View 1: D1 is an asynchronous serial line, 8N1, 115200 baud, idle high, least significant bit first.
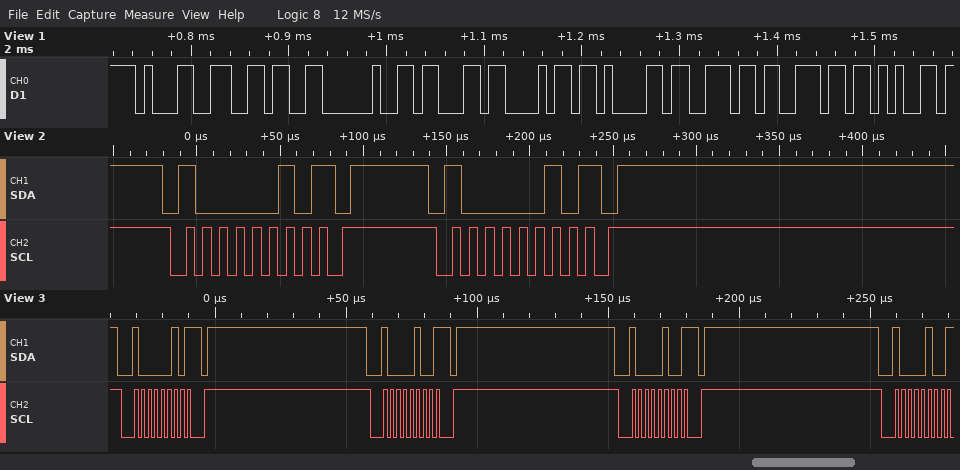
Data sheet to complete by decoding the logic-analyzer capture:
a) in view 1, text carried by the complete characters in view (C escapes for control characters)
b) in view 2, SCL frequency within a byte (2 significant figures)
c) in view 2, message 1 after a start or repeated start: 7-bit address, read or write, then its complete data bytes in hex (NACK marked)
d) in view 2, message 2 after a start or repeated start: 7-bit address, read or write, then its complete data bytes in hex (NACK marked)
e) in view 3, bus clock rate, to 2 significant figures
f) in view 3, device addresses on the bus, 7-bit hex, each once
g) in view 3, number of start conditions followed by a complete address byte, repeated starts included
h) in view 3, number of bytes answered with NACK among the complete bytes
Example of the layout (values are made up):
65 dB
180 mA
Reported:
"16 channe"
100 kHz
0x41 write NACK
0x41 write NACK
400 kHz
0x41 0x42
4
4
